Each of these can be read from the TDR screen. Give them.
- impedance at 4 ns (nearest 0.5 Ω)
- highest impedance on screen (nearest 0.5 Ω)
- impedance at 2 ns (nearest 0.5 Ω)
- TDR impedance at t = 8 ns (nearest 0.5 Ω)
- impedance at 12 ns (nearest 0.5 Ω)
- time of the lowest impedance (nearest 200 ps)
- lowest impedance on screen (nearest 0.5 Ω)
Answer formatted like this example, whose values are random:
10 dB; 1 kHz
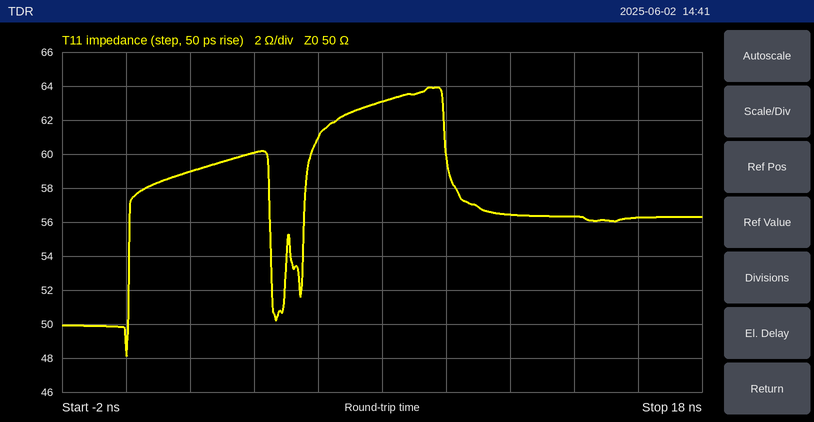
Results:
60.0 Ω; 64.0 Ω; 59.0 Ω; 63.0 Ω; 56.5 Ω; 0.0 ns; 48.0 Ω
